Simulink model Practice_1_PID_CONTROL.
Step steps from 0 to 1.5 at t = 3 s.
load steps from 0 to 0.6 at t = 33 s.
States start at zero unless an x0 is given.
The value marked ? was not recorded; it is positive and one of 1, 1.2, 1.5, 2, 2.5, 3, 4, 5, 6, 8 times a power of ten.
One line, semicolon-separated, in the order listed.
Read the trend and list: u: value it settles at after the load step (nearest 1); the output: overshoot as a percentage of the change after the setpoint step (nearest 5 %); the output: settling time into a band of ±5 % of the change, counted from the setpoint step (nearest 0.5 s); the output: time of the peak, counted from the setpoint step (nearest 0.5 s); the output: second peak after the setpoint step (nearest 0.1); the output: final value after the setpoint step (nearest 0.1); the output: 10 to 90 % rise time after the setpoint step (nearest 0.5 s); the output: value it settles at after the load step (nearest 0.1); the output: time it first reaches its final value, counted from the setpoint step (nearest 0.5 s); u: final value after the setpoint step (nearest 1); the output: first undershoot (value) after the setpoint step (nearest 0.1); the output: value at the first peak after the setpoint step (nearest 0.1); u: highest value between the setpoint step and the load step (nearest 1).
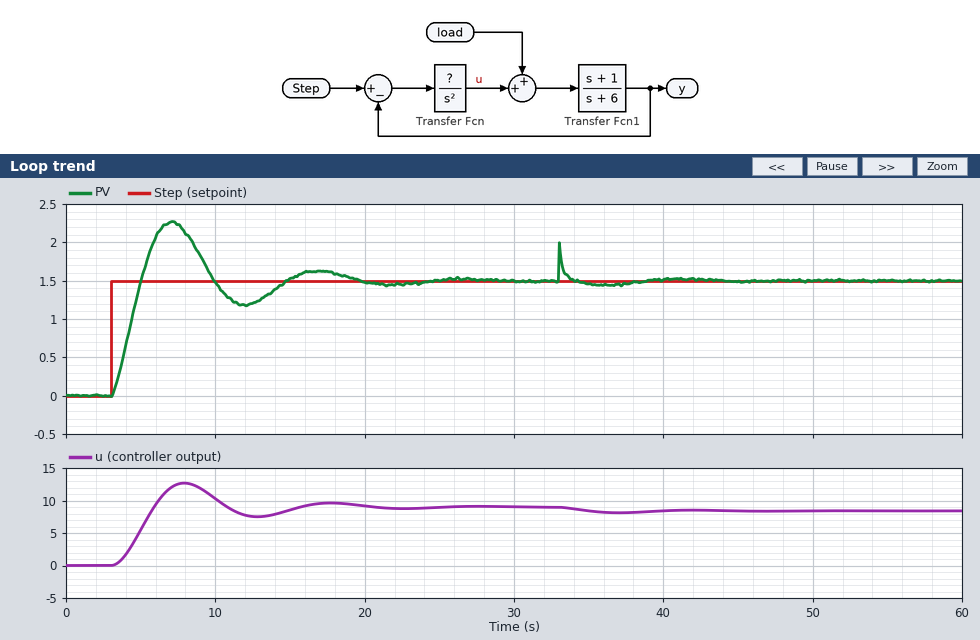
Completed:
8; 50 %; 15.5 s; 4.0 s; 1.6; 1.5; 1.5 s; 1.5; 2.0 s; 9; 1.2; 2.3; 13
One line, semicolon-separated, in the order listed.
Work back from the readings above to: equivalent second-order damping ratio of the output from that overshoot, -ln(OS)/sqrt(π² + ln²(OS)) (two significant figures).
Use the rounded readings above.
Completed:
0.22
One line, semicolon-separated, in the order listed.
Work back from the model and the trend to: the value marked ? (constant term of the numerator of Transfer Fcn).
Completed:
2.5
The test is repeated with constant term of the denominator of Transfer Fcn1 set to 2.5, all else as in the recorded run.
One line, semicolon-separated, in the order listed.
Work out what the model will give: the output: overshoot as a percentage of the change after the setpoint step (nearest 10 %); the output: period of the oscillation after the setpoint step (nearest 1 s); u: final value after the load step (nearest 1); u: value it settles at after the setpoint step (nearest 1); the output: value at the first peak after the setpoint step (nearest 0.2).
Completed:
60 %; 6 s; 3; 4; 2.4
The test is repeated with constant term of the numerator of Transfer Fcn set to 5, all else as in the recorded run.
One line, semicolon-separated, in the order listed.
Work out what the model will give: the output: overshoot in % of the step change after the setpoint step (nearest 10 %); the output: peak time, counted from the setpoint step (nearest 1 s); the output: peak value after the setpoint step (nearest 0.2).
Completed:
40 %; 3 s; 2.2
